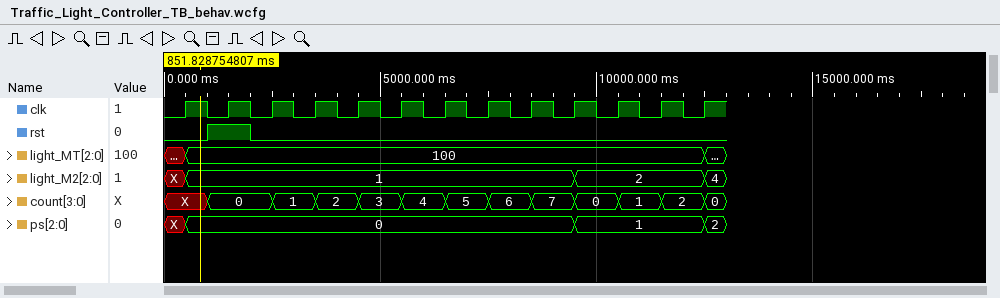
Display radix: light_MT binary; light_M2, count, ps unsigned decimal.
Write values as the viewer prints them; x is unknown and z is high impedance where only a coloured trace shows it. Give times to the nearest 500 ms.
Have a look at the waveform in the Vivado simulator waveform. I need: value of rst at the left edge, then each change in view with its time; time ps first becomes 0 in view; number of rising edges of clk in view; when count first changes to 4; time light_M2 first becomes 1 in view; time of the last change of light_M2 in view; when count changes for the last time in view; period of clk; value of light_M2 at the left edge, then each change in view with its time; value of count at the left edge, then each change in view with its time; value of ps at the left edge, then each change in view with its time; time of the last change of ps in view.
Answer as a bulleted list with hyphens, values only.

- 0, 1 at 1000 ms, 0 at 2000 ms
- 500 ms
- 13
- 5500 ms
- 500 ms
- 12500 ms
- 12500 ms
- 1000 ms
- X, 1 at 500 ms, 2 at 9500 ms, 4 at 12500 ms
- X, 0 at 1000 ms, 1 at 2500 ms, 2 at 3500 ms, 3 at 4500 ms, 4 at 5500 ms, 5 at 6500 ms, 6 at 7500 ms, 7 at 8500 ms, 0 at 9500 ms, 1 at 10500 ms, 2 at 11500 ms, 0 at 12500 ms
- X, 0 at 500 ms, 1 at 9500 ms, 2 at 12500 ms
- 12500 ms
